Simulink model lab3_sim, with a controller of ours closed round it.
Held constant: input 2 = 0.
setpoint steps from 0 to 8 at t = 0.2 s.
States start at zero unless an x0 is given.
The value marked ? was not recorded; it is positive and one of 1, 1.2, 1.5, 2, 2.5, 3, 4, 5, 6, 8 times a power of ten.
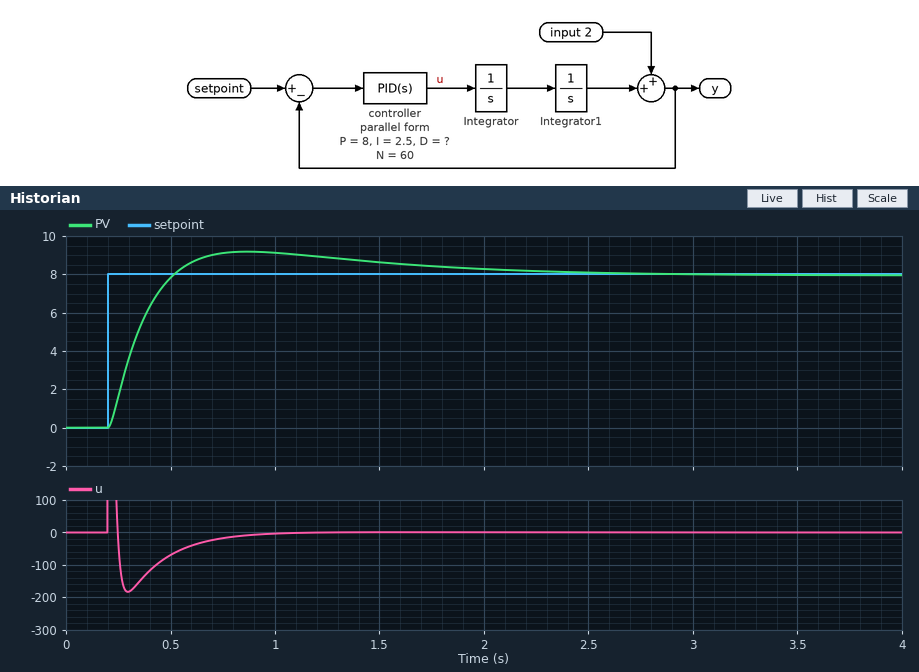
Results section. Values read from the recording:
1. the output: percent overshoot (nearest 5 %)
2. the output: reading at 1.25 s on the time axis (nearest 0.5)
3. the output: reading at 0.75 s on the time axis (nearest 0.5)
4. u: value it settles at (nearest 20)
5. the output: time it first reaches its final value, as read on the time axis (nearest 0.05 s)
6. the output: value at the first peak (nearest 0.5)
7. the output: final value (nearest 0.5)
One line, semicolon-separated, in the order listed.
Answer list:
15 %; 9.0; 9.0; 0; 0.50 s; 9.0; 8.0
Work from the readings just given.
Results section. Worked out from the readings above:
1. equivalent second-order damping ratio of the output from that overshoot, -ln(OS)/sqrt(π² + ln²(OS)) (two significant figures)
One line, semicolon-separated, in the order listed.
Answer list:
0.52
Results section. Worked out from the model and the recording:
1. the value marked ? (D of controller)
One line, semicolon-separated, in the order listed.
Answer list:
6
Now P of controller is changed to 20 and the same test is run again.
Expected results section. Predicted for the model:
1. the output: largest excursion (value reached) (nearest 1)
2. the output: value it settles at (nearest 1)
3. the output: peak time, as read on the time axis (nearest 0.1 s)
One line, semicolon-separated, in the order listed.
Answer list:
10; 8; 0.7 s
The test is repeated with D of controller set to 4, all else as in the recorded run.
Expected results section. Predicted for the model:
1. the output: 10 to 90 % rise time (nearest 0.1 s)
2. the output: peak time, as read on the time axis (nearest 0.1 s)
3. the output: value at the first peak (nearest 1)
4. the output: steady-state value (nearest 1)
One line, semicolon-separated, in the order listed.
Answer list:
0.3 s; 1.0 s; 10; 8
